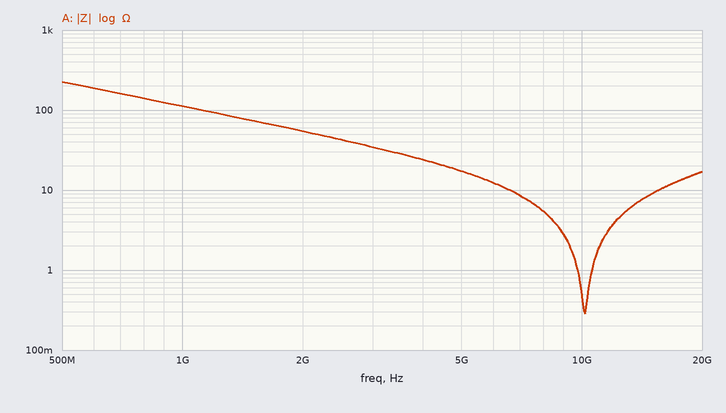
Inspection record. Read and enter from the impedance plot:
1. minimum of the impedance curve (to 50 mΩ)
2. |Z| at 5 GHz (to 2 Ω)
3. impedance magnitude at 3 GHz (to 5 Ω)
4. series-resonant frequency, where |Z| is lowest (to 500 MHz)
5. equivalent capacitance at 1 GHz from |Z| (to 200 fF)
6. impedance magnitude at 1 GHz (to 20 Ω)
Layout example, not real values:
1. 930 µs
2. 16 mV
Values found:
1. 300 mΩ
2. 18 Ω
3. 35 Ω
4. 10.0 GHz
5. 1.4 pF
6. 120 Ω
